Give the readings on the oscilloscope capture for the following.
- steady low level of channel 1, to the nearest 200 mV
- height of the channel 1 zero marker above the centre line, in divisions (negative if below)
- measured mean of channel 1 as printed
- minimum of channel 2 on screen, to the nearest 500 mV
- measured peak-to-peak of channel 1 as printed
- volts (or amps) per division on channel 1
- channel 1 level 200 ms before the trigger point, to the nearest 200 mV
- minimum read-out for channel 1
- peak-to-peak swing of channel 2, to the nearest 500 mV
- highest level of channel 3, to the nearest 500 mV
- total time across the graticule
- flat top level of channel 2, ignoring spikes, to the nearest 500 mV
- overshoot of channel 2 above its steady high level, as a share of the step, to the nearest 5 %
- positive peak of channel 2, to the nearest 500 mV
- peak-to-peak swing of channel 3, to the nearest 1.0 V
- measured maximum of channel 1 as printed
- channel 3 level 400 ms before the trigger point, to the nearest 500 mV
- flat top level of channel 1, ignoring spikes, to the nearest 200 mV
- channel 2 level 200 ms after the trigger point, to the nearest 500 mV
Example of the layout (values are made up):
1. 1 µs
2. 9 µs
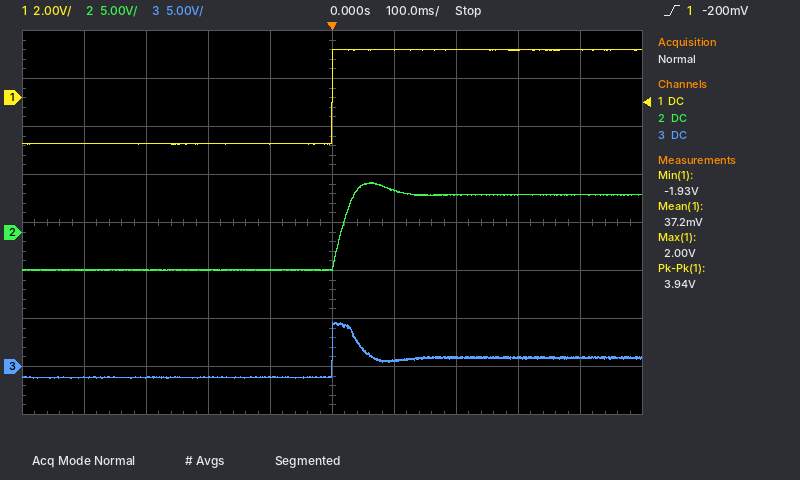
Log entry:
1. -2.0 V
2. +2.6 div
3. 37.2 mV
4. -4.0 V
5. 3.94 V
6. 2 V
7. -2.0 V
8. -1.93 V
9. 9.0 V
10. 4.5 V
11. 1 s
12. 4.0 V
13. 15 %
14. 5.0 V
15. 6.0 V
16. 2.00 V
17. -1.0 V
18. 2.0 V
19. 4.0 V
